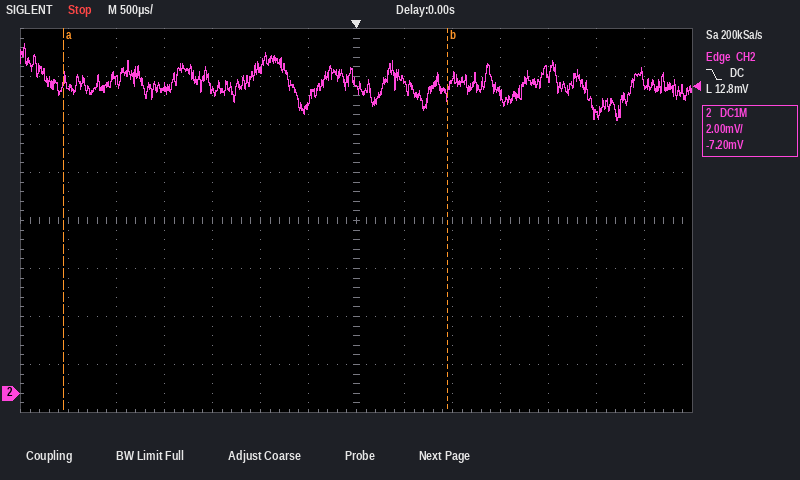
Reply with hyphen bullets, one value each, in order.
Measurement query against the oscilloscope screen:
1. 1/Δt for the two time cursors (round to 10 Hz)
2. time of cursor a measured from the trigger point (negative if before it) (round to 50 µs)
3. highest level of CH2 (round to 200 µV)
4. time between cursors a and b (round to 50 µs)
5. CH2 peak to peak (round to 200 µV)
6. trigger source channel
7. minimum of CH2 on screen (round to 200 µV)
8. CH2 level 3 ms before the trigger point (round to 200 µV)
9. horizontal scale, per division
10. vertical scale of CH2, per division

- 250 Hz
- -3.05 ms
- 14.6 mV
- 4.00 ms
- 3.2 mV
- CH2
- 11.4 mV
- 12.8 mV
- 500 µs
- 2 mV
